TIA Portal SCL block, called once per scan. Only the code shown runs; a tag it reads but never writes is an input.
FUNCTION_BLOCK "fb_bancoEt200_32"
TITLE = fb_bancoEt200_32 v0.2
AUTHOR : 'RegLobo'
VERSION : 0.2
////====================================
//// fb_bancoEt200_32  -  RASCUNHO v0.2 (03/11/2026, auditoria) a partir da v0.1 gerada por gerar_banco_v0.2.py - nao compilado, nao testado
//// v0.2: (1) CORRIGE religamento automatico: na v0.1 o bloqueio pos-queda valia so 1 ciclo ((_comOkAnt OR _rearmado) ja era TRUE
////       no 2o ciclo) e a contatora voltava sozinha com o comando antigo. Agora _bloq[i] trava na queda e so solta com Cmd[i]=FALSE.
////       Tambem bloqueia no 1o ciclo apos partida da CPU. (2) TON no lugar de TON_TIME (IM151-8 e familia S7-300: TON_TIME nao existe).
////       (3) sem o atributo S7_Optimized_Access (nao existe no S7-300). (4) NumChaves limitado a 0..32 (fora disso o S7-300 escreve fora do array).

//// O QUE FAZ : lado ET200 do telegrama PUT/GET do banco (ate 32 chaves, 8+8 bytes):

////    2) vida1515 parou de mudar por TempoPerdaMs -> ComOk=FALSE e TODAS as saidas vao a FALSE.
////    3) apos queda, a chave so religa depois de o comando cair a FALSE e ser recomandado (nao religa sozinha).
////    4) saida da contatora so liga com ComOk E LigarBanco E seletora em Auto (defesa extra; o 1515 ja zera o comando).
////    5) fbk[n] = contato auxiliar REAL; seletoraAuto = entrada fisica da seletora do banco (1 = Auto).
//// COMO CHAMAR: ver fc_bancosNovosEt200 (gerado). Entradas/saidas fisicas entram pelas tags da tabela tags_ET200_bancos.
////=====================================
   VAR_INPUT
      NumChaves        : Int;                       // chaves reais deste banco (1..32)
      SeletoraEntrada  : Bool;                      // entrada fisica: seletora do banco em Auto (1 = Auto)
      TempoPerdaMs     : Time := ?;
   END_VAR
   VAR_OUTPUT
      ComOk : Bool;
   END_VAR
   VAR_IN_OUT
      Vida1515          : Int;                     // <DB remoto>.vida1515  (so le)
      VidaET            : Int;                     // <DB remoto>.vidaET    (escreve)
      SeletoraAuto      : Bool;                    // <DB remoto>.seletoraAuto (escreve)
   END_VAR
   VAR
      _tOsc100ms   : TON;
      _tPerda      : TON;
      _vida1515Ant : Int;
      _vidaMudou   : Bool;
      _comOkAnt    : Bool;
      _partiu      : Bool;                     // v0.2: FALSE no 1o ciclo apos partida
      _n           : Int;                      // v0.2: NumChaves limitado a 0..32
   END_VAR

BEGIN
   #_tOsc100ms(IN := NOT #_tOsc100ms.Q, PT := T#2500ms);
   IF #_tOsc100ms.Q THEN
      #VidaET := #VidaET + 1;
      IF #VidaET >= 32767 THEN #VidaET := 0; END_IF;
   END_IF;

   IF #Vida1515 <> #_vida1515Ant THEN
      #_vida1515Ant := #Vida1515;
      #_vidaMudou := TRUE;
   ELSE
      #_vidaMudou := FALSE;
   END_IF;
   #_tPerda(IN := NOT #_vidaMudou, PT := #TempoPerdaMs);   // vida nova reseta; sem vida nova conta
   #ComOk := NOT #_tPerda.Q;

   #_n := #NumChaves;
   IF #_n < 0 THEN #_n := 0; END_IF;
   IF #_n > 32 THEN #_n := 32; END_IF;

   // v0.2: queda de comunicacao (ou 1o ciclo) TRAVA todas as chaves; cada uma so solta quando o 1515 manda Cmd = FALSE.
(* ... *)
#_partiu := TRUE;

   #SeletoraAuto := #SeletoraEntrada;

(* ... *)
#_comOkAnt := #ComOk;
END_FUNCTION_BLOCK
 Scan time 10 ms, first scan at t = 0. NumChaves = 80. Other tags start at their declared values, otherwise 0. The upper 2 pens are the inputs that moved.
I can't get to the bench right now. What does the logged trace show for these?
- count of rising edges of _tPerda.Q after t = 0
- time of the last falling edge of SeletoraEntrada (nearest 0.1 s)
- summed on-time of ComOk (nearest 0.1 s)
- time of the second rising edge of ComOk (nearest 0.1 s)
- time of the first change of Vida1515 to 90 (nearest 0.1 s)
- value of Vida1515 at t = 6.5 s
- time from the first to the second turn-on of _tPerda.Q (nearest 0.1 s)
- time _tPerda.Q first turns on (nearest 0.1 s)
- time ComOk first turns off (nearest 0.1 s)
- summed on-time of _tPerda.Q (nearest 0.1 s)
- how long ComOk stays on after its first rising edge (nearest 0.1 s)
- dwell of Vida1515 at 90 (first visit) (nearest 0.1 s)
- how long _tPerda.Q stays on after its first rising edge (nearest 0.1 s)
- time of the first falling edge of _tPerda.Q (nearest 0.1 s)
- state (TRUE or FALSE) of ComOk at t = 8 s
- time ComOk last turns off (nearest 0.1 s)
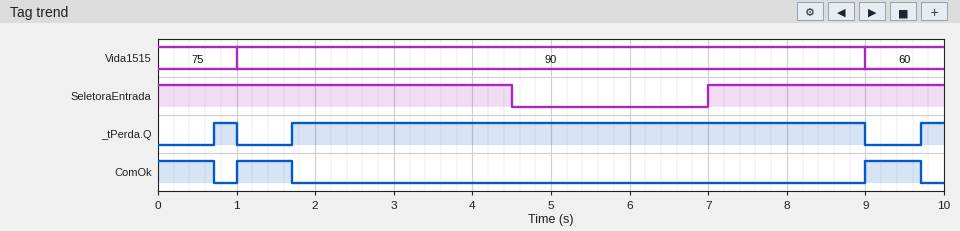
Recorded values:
3
4.5 s
2.1 s
9.0 s
1.0 s
90
1.0 s
0.7 s
0.7 s
7.9 s
0.7 s
8.0 s
0.3 s
1.0 s
FALSE
9.7 s
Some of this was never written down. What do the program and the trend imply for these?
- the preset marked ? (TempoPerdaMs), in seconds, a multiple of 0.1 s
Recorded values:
0.7 s
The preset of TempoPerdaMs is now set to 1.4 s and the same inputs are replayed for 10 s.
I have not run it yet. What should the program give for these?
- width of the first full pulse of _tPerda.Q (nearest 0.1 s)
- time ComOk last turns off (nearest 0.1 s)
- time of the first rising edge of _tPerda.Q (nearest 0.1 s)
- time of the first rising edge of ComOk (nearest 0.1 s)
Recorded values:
6.6 s
2.4 s
2.4 s
9.0 s
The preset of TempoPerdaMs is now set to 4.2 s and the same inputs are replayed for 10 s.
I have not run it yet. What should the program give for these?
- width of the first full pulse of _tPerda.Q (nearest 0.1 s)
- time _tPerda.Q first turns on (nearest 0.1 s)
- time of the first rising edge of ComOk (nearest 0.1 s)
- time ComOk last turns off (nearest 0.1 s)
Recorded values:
3.8 s
5.2 s
9.0 s
5.2 s
